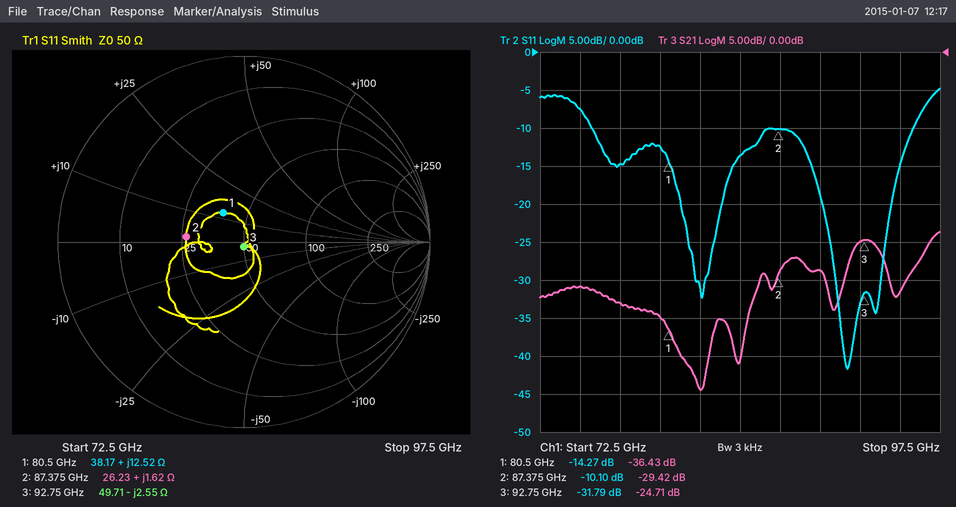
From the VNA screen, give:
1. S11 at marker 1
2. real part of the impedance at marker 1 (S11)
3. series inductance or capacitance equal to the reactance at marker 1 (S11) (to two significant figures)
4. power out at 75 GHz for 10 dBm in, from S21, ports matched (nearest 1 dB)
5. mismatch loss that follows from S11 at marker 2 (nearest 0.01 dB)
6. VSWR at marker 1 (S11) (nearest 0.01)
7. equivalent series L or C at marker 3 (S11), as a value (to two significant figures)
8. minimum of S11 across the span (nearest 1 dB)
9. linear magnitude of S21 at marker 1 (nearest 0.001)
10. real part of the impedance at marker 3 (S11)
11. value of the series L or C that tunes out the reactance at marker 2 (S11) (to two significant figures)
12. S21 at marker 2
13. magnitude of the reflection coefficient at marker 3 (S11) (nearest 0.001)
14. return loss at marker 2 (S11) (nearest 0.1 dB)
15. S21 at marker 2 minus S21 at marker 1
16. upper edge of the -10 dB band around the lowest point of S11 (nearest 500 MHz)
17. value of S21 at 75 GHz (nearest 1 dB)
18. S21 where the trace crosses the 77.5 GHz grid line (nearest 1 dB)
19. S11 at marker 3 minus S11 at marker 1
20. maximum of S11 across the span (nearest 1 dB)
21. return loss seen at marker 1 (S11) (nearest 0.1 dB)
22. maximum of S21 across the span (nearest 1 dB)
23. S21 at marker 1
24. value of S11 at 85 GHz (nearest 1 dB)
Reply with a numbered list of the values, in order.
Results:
1. -14.27 dB
2. 38.17 Ω
3. 25 pH
4. -21 dBm
5. 0.45 dB
6. 1.48
7. 670 fF
8. -42 dB
9. 0.015
10. 49.71 Ω
11. 1.1 pF
12. -29.42 dB
13. 0.026
14. 10.1 dB
15. 7.01 dB
16. 96.0 GHz
17. -31 dB
18. -33 dB
19. -17.52 dB
20. -5 dB
21. 14.3 dB
22. -24 dB
23. -36.43 dB
24. -14 dB
